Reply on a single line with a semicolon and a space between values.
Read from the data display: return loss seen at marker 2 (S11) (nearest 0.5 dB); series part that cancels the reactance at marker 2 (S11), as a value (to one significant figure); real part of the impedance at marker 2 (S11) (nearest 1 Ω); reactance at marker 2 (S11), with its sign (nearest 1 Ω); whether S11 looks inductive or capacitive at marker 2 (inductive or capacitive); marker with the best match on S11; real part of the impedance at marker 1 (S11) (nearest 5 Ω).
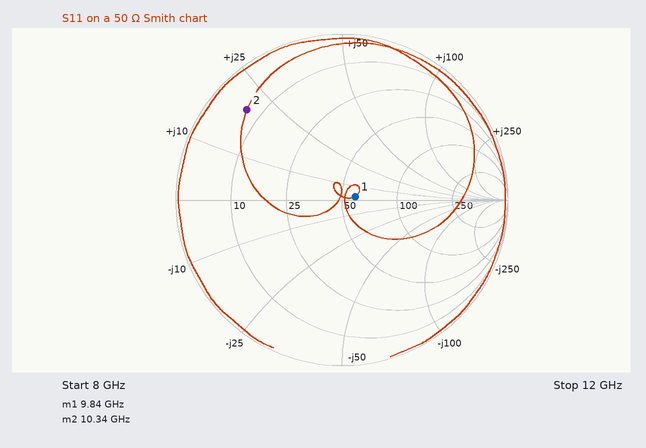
2.0 dB; 800 fF; 7 Ω; +20 Ω; inductive; marker 1; 60 Ω
